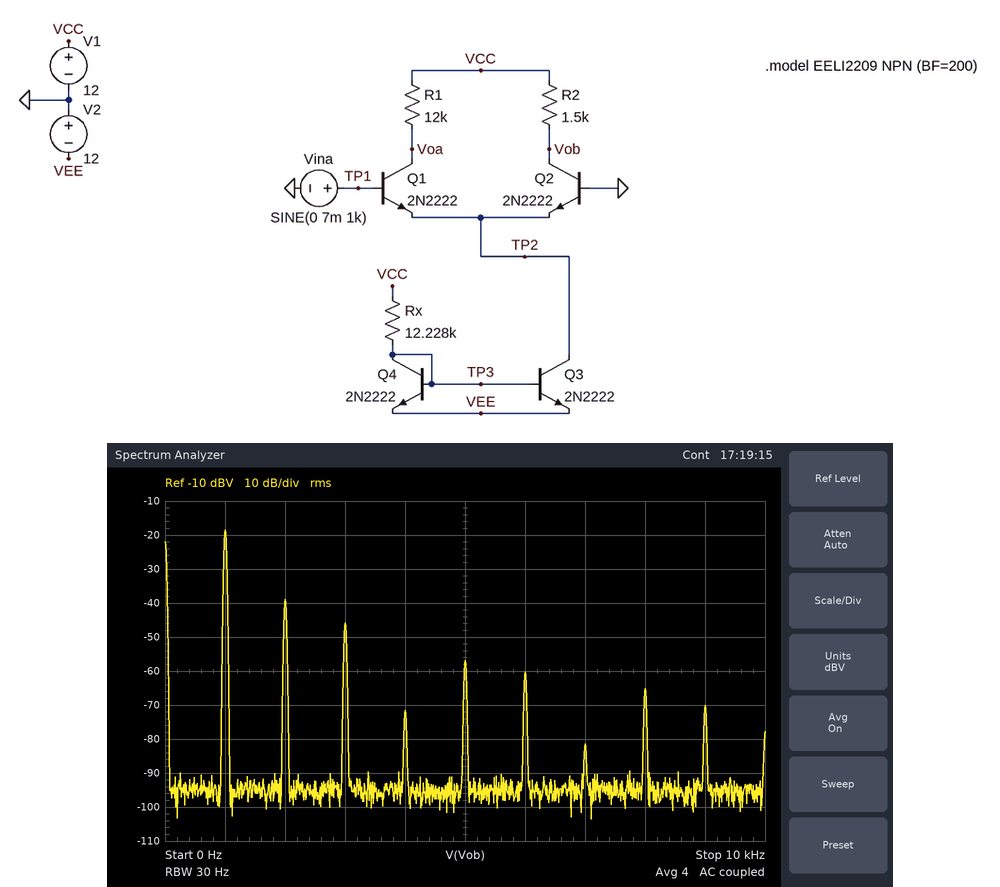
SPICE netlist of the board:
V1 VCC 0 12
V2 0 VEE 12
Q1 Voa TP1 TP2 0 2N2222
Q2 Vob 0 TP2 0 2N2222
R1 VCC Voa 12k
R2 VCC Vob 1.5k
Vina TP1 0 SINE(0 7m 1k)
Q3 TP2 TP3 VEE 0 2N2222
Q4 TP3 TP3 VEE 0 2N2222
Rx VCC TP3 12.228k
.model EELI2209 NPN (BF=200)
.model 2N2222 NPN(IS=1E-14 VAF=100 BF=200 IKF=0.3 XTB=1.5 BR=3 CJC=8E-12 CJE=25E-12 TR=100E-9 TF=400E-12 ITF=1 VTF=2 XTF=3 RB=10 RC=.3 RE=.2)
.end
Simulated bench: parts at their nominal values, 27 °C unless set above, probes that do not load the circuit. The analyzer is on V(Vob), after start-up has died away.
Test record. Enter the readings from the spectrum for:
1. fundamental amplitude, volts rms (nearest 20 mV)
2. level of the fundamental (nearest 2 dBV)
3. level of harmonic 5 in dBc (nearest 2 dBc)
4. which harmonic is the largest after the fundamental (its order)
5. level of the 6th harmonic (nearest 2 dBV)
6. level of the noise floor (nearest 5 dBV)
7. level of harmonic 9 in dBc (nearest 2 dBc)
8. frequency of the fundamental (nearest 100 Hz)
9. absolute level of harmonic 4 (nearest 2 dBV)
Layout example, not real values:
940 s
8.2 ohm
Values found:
120 mV
-18 dBV
-38 dBc
2
-60 dBV
-95 dBV
-52 dBc
1.0 kHz
-72 dBV
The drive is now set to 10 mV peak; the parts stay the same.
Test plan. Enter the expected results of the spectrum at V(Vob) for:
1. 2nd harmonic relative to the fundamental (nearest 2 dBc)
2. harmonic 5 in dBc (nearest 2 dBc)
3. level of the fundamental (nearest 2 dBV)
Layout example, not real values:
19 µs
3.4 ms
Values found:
-18 dBc
-36 dBc
-16 dBV
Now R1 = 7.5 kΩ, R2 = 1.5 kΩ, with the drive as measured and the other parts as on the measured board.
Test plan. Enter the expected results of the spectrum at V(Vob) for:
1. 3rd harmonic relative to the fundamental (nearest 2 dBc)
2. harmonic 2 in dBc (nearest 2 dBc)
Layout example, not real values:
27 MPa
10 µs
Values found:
-58 dBc
-56 dBc
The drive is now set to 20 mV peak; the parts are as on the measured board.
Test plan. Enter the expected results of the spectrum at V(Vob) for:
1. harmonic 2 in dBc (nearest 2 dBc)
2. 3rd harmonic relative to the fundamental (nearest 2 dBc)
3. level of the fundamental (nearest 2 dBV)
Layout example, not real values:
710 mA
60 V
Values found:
-18 dBc
-32 dBc
-10 dBV
